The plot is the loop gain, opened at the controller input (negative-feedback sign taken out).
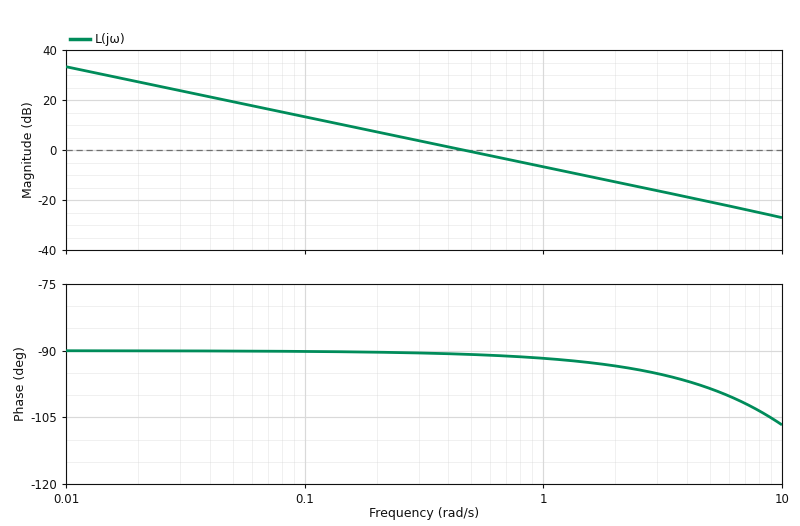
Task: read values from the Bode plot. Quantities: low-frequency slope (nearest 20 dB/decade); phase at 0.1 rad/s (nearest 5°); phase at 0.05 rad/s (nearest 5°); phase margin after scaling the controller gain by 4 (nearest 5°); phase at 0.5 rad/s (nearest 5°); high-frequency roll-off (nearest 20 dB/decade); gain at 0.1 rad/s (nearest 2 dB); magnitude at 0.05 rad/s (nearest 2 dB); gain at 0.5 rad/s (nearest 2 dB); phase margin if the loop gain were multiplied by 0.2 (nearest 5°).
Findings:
-20 dB/decade
-90°
-90°
85°
-90°
-20 dB/decade
14 dB
20 dB
0 dB
90°
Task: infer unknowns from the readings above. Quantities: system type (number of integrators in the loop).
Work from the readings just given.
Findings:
1
